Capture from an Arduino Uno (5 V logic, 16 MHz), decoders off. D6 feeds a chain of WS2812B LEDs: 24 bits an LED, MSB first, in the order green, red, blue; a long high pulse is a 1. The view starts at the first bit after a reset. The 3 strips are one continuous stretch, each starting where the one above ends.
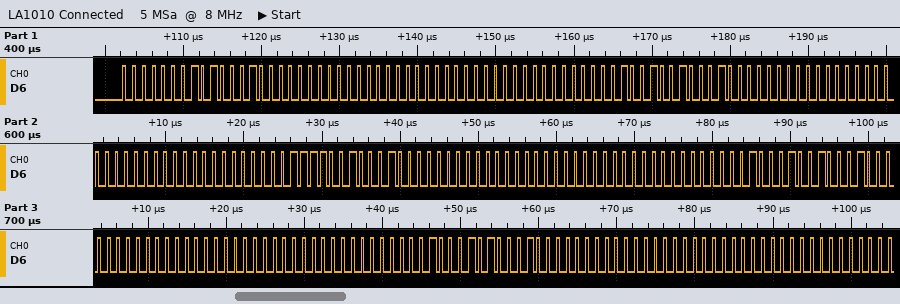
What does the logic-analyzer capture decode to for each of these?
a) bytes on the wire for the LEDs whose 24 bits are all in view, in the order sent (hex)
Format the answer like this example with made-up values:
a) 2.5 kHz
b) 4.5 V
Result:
a) 01 44 00 00 00 00 12 44 00 00 00 00 1E 44 00 00 00 00 22 44 00 00 00 00 11 44 00 00 00 00
